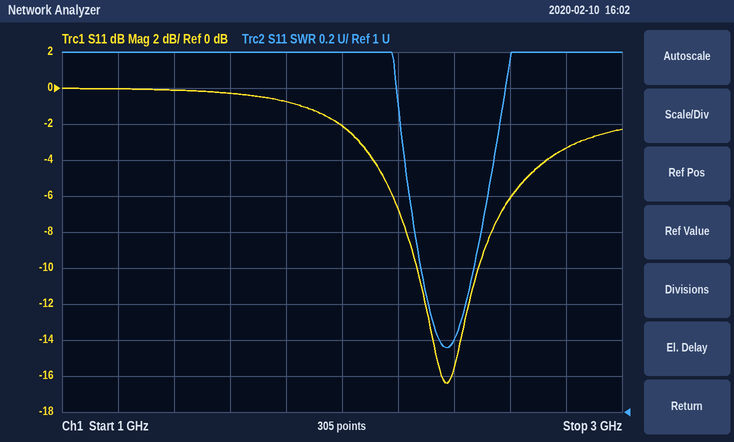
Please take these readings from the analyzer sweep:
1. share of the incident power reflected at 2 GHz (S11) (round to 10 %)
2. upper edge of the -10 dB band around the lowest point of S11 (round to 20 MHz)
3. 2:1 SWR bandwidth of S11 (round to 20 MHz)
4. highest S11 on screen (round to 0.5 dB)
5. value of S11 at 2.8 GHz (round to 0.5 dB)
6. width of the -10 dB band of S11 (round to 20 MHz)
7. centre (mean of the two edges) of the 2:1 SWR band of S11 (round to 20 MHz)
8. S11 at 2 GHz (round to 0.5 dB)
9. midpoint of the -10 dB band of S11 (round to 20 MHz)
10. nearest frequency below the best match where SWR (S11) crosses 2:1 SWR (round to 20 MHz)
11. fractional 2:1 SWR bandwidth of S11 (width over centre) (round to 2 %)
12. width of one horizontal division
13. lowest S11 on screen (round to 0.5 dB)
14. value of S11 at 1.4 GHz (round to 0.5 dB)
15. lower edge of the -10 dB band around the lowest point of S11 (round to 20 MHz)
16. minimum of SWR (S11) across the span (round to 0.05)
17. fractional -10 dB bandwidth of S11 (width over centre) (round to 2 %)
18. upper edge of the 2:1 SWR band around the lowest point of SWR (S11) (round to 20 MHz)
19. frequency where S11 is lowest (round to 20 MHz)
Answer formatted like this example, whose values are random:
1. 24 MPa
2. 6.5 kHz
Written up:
1. 60 %
2. 2.48 GHz
3. 240 MHz
4. 0.0 dB
5. -3.5 dB
6. 220 MHz
7. 2.38 GHz
8. -2.0 dB
9. 2.38 GHz
10. 2.26 GHz
11. 10 %
12. 200 MHz
13. -16.5 dB
14. 0.0 dB
15. 2.26 GHz
16. 1.35
17. 10 %
18. 2.50 GHz
19. 2.38 GHz
